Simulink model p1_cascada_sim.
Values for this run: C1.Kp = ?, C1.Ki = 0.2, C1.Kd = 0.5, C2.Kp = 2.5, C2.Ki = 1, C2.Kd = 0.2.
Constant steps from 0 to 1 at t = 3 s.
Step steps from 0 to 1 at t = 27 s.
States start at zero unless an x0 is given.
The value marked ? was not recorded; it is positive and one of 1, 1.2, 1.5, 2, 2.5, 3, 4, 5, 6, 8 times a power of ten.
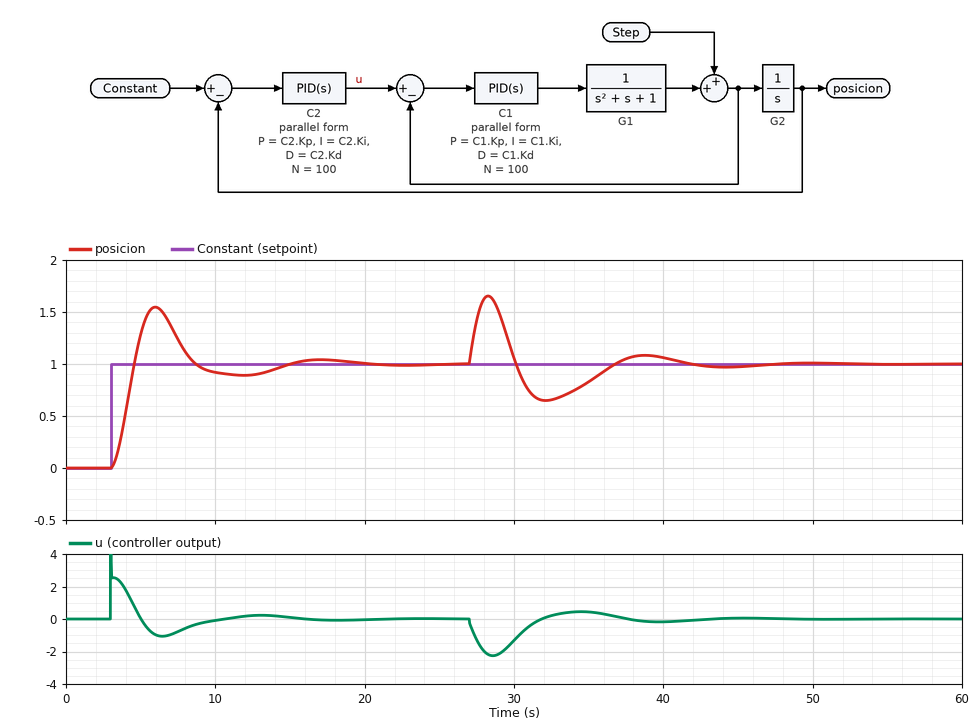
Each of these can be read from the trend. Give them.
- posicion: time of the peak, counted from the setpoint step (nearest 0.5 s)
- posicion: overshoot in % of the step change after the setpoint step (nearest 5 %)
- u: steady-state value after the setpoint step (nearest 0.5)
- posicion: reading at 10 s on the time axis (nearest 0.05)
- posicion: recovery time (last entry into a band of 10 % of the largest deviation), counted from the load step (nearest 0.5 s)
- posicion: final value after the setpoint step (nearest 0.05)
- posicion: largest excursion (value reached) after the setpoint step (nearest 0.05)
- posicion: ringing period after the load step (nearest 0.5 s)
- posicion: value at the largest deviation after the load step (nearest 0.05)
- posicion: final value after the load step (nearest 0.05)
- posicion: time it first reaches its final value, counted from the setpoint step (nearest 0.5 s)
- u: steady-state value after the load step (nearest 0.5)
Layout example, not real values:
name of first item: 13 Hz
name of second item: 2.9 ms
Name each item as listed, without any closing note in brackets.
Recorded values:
posicion: time of the peak, counted from the setpoint step: 3.0 s
posicion: overshoot in % of the step change after the setpoint step: 55 %
u: steady-state value after the setpoint step: 0.0
posicion: reading at 10 s on the time axis: 0.90
posicion: recovery time (last entry into a band of 10 % of the largest deviation), counted from the load step: 13.0 s
posicion: final value after the setpoint step: 1.00
posicion: largest excursion (value reached) after the setpoint step: 1.55
posicion: ringing period after the load step: 10.5 s
posicion: value at the largest deviation after the load step: 1.65
posicion: final value after the load step: 1.00
posicion: time it first reaches its final value, counted from the setpoint step: 1.5 s
u: steady-state value after the load step: 0.0
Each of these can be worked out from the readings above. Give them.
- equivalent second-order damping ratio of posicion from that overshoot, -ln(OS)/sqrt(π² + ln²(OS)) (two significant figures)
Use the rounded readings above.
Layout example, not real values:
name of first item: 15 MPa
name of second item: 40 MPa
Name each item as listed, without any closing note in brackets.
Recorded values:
equivalent second-order damping ratio of posicion from that overshoot, -ln(OS)/sqrt(π² + ln²(OS)): 0.19
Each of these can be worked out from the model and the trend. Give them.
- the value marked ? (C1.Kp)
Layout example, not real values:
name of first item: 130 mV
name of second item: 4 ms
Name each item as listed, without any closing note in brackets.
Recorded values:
the value marked ?: 0.4
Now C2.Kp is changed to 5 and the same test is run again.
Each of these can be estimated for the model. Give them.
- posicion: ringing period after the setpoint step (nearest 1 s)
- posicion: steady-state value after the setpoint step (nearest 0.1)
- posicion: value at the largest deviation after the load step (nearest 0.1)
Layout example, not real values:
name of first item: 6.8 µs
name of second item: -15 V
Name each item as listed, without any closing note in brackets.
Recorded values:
posicion: ringing period after the setpoint step: 4 s
posicion: steady-state value after the setpoint step: 1.0
posicion: value at the largest deviation after the load step: 1.5
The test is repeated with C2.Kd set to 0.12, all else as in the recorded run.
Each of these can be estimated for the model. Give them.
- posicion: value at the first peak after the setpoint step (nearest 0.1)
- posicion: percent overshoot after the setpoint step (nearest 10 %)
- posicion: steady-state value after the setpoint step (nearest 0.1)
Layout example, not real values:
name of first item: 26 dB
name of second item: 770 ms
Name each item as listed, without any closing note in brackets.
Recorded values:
posicion: value at the first peak after the setpoint step: 1.6
posicion: percent overshoot after the setpoint step: 60 %
posicion: steady-state value after the setpoint step: 1.0
